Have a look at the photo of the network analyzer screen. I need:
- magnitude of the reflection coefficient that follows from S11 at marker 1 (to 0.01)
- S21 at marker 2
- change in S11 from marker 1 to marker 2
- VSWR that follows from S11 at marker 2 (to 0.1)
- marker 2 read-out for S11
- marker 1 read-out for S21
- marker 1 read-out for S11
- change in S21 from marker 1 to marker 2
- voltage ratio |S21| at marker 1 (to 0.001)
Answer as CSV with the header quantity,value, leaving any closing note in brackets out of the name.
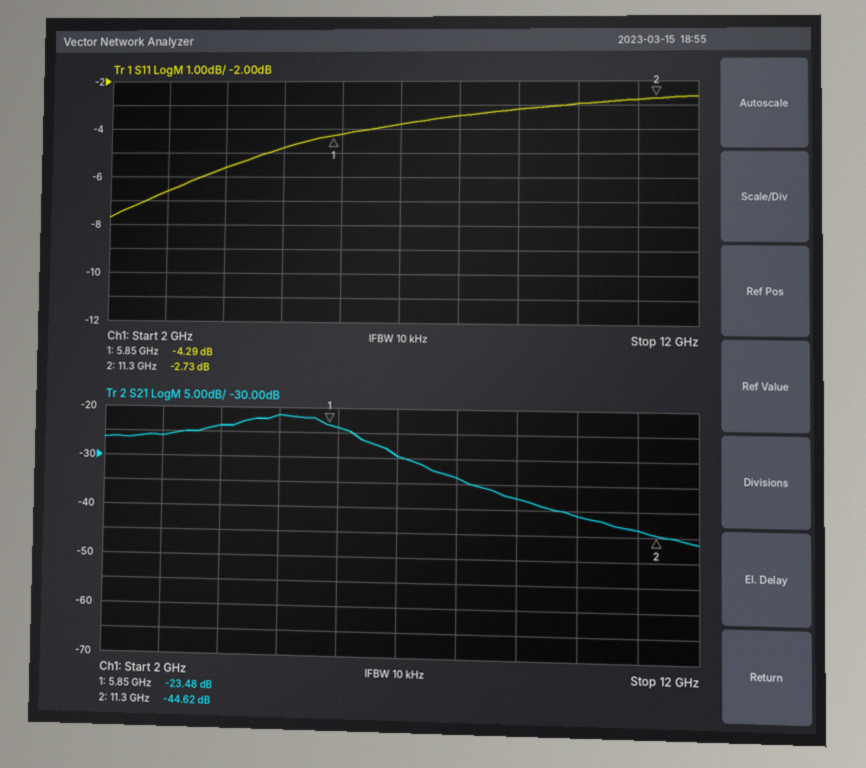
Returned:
quantity,value
magnitude of the reflection coefficient that follows from S11 at marker 1,0.61
S21 at marker 2,-44.62 dB
change in S11 from marker 1 to marker 2,1.56 dB
VSWR that follows from S11 at marker 2,6.4
marker 2 read-out for S11,-2.73 dB
marker 1 read-out for S21,-23.48 dB
marker 1 read-out for S11,-4.29 dB
change in S21 from marker 1 to marker 2,-21.14 dB
voltage ratio |S21| at marker 1,0.067
